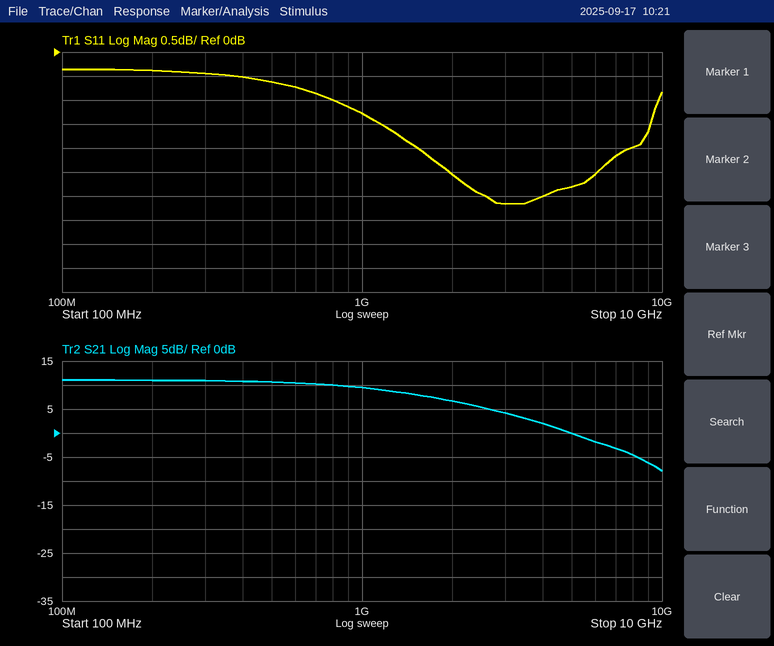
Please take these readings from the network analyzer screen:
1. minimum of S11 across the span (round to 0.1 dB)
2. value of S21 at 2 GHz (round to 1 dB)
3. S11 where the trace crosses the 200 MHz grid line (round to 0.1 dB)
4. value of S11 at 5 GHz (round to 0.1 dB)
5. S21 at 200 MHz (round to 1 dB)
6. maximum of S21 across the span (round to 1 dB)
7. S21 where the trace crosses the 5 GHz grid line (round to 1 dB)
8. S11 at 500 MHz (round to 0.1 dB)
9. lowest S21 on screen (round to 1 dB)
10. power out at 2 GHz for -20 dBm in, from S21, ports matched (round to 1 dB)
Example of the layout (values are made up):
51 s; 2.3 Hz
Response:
-3.2 dB; 7 dB; -0.4 dB; -2.8 dB; 11 dB; 11 dB; 0 dB; -0.6 dB; -8 dB; -13 dBm
